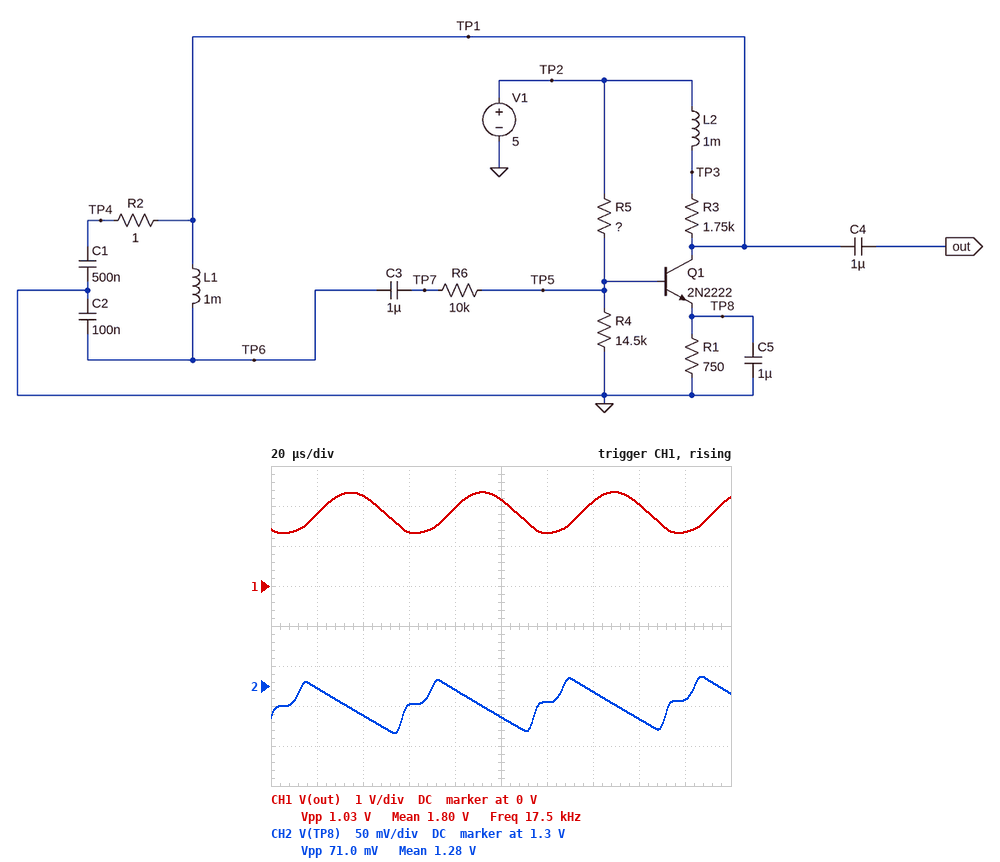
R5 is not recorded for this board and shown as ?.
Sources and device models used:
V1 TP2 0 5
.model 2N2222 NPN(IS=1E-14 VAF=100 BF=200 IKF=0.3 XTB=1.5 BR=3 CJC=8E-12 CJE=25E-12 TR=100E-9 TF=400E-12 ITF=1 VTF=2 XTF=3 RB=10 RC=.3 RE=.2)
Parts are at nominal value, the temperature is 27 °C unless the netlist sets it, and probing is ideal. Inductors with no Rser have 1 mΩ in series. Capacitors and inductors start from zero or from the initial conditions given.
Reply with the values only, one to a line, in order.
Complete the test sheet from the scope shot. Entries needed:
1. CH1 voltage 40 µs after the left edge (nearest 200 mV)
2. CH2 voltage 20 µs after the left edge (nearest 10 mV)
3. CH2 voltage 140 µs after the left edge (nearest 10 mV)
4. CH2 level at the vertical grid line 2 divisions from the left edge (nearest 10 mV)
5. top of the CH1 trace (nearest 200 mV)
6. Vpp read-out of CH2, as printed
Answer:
2.2 V
1.30 V
1.29 V
1.26 V
2.4 V
71.0 mV
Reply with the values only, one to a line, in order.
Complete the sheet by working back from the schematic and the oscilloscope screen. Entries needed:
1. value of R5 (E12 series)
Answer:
82 kΩ
